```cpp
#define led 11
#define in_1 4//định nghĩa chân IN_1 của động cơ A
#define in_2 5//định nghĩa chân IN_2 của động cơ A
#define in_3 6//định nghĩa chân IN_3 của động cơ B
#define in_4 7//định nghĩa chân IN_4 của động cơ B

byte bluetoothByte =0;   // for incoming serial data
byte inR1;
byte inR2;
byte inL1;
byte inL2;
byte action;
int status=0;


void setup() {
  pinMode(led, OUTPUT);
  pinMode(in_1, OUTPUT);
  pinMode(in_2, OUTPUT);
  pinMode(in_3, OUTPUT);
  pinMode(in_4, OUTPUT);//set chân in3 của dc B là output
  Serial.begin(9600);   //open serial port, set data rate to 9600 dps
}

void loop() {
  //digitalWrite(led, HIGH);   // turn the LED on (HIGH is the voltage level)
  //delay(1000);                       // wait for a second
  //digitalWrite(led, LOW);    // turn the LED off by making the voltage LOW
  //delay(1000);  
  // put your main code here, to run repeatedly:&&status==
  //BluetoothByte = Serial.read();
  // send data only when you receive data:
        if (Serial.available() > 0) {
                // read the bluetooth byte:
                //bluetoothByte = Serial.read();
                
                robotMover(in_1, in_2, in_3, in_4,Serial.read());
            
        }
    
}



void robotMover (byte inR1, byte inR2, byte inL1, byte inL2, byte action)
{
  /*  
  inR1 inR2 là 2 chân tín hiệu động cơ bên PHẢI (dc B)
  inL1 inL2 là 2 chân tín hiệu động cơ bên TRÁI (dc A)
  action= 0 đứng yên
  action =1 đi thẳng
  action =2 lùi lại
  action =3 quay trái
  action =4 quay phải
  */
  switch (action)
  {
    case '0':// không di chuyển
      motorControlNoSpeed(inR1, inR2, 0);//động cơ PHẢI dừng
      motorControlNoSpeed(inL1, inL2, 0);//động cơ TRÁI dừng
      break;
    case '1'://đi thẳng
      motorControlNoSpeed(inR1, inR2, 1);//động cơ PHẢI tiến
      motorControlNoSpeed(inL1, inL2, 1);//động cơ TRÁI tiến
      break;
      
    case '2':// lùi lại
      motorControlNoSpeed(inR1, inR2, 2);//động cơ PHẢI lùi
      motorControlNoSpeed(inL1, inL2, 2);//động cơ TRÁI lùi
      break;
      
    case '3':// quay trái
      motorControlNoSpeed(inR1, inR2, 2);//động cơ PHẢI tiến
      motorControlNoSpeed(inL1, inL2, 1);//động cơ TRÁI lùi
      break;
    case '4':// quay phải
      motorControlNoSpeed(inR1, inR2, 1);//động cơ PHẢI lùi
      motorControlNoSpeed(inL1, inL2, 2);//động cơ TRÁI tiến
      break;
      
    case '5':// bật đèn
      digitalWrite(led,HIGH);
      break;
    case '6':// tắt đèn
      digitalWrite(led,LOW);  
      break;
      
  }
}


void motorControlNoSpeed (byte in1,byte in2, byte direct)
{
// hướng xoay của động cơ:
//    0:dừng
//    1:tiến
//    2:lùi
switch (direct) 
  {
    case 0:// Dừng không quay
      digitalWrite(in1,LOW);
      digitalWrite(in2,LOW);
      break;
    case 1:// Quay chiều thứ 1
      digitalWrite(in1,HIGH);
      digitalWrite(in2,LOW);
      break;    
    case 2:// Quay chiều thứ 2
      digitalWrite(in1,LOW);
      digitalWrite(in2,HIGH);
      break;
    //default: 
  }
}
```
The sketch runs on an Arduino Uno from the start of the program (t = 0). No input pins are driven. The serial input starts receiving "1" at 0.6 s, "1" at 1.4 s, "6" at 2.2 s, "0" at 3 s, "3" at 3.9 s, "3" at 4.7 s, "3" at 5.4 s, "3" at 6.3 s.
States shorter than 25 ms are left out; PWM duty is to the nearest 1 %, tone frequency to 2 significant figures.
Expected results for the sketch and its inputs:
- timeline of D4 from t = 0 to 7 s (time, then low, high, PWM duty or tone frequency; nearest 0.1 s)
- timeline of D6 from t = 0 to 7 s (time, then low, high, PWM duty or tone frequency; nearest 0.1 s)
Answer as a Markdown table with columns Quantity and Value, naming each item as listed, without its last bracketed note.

| Quantity | Value |
|---|---|
| timeline of D4 from t = 0 to 7 s | 0 s low; 0.6 s high; 3 s low |
| timeline of D6 from t = 0 to 7 s | 0 s low; 0.6 s high; 3 s low; 3.9 s high |
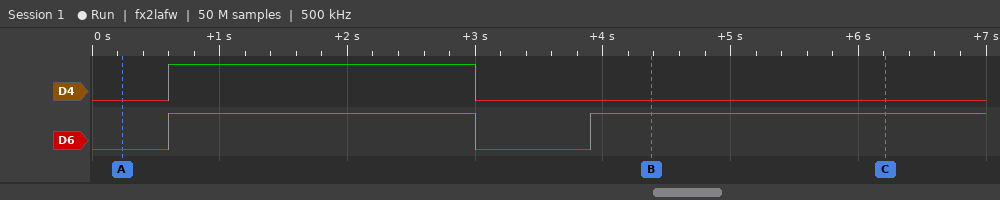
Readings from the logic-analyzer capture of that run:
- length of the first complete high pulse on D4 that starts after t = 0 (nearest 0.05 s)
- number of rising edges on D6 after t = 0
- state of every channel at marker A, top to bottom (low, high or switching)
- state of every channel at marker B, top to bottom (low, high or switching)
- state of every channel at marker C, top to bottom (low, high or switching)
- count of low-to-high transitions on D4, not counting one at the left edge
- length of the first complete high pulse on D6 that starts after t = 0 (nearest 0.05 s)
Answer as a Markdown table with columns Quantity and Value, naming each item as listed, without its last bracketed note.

| Quantity | Value |
|---|---|
| length of the first complete high pulse on D4 that starts after t = 0 | 2.40 s |
| number of rising edges on D6 after t = 0 | 2 |
| state of every channel at marker A, top to bottom | D4 low, D6 low |
| state of every channel at marker B, top to bottom | D4 low, D6 high |
| state of every channel at marker C, top to bottom | D4 low, D6 high |
| count of low-to-high transitions on D4, not counting one at the left edge | 1 |
| length of the first complete high pulse on D6 that starts after t = 0 | 2.40 s |
